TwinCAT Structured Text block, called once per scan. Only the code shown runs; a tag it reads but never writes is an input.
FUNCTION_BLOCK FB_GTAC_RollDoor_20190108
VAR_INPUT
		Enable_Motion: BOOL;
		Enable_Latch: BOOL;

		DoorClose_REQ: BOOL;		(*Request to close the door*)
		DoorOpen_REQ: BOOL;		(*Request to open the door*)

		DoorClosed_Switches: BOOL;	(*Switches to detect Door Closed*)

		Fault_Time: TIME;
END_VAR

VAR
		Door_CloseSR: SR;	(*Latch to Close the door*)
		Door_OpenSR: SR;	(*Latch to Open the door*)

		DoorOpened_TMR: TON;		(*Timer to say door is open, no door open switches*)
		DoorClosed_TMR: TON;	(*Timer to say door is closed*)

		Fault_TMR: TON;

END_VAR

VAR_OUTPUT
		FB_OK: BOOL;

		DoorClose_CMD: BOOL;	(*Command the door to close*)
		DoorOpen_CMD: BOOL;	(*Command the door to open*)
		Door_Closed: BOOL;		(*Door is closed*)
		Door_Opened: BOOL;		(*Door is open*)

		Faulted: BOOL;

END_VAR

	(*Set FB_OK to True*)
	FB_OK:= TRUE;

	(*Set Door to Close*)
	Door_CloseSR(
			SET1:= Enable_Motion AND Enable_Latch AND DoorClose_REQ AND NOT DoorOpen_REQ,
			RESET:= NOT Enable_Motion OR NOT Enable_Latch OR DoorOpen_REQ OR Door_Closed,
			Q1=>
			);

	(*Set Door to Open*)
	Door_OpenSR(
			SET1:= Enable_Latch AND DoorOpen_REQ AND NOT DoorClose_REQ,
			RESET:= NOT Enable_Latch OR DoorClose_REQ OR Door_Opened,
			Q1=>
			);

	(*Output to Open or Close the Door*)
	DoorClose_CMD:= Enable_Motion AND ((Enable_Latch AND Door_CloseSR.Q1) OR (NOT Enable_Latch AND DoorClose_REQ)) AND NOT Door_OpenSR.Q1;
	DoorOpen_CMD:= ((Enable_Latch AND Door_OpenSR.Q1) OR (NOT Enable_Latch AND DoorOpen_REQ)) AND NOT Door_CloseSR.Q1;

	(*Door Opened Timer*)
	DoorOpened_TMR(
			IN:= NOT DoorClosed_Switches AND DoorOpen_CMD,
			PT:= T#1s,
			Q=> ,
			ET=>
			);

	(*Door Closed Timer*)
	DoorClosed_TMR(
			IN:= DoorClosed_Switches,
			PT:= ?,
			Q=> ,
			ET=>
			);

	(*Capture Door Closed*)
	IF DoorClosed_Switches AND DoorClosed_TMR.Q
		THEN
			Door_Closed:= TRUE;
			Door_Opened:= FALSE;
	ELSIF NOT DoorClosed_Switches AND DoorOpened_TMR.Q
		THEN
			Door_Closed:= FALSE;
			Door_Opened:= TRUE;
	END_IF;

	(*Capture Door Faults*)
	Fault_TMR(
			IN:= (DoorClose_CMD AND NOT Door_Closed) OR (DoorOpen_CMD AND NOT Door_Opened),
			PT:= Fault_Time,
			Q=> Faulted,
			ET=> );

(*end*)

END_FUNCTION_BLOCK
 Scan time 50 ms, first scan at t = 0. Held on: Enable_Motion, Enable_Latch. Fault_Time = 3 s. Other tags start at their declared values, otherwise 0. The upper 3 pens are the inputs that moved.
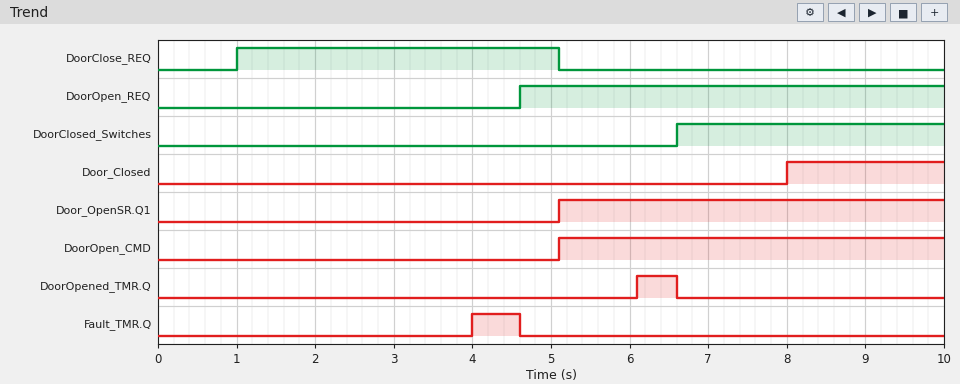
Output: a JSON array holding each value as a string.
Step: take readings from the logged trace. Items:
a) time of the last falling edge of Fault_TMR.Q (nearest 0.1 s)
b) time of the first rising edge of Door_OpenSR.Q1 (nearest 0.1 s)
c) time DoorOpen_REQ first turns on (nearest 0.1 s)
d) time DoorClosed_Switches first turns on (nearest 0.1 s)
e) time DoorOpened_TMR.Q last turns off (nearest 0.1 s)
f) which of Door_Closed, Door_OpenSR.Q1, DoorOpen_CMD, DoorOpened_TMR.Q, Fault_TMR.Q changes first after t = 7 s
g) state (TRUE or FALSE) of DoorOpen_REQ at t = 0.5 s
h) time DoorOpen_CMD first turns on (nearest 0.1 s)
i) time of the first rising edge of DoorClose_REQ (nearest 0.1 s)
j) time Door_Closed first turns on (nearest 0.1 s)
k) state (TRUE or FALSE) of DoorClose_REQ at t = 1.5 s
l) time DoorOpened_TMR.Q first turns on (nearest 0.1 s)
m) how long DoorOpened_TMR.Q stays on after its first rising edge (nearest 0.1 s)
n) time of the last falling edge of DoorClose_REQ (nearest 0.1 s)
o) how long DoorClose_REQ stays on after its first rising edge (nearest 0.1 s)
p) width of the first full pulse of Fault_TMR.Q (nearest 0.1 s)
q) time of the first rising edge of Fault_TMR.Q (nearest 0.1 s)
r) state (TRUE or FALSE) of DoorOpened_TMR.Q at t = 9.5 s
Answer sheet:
["4.6 s", "5.1 s", "4.6 s", "6.6 s", "6.6 s", "Door_Closed", "FALSE", "5.1 s", "1.0 s", "8.0 s", "TRUE", "6.1 s", "0.5 s", "5.1 s", "4.1 s", "0.6 s", "4.0 s", "FALSE"]
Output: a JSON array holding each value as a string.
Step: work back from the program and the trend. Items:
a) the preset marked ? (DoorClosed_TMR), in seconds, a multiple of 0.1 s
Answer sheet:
["1.4 s"]
